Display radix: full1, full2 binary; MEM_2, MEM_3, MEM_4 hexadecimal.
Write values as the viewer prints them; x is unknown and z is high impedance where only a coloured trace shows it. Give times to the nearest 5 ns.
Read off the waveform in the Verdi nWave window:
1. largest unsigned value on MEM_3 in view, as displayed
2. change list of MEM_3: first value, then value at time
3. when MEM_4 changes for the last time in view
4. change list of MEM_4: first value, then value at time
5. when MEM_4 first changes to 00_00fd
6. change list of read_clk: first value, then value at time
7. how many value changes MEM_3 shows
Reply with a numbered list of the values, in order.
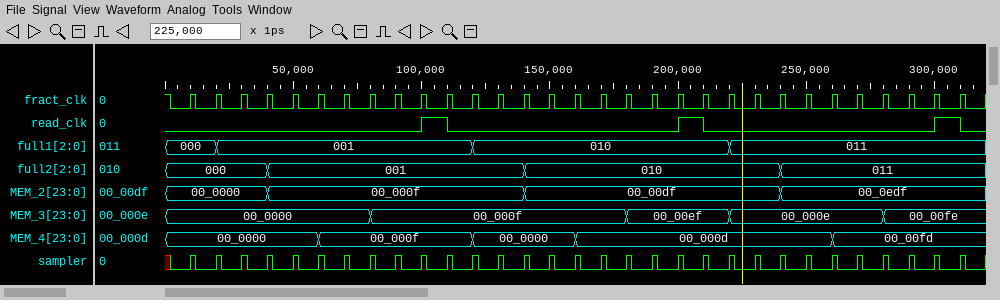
1. 00_00fe
2. 00_0000, 00_000f at 80 ns, 00_00ef at 180 ns, 00_000e at 220 ns, 00_00fe at 280 ns
3. 260 ns
4. 00_0000, 00_000f at 60 ns, 00_0000 at 120 ns, 00_000d at 160 ns, 00_00fd at 260 ns
5. 260 ns
6. 0, 1 at 100 ns, 0 at 110 ns, 1 at 200 ns, 0 at 210 ns, 1 at 300 ns, 0 at 310 ns
7. 4
